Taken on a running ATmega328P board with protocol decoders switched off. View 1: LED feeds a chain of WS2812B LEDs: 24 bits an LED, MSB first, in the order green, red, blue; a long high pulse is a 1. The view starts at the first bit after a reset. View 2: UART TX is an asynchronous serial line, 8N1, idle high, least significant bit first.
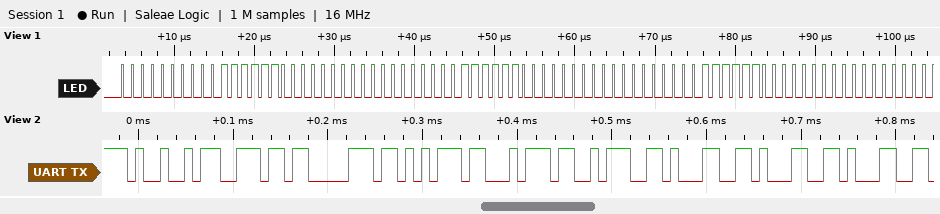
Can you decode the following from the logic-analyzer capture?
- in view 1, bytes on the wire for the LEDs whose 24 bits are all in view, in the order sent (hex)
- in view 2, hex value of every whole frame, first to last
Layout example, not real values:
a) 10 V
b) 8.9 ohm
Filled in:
a) 00 3F 00 00 3F 00 00 3F 00
b) 49 6E 70 75 74 3A 31 31 31
